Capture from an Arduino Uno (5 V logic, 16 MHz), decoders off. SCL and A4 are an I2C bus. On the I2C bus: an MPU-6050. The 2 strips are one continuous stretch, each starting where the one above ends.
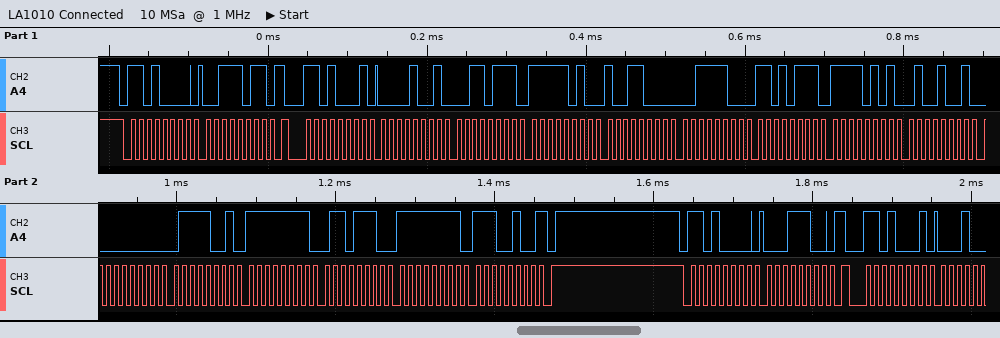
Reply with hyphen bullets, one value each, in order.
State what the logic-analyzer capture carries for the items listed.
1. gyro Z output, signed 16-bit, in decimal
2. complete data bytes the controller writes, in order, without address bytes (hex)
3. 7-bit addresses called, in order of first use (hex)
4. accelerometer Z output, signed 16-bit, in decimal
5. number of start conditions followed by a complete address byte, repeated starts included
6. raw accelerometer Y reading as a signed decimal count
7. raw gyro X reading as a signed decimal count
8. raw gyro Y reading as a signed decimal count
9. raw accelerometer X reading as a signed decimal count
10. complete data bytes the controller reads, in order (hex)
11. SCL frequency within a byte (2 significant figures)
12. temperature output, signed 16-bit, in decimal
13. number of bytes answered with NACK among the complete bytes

- -28
- 3B 1C
- 0x68
- 15575
- 4
- -1384
- 121
- -146
- 2359
- 09 37 FA 98 3C D7 F5 49 00 79 FF 6E FF E4
- 100 kHz
- -2743
- 1
